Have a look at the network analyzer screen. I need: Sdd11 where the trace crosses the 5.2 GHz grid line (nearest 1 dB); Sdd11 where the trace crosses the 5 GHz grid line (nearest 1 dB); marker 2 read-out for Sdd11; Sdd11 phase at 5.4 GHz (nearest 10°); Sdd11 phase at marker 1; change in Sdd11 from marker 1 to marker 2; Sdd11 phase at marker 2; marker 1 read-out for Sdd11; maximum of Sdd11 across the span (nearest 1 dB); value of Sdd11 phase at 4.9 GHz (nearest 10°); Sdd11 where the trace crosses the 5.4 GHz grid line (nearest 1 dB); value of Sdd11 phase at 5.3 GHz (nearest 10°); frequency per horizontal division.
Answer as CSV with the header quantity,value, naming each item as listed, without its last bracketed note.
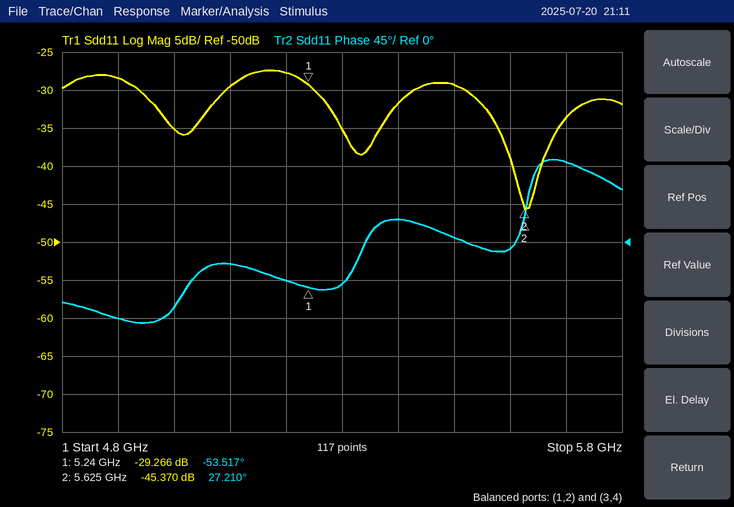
quantity,value
Sdd11 where the trace crosses the 5.2 GHz grid line,-28 dB
Sdd11 where the trace crosses the 5 GHz grid line,-35 dB
marker 2 read-out for Sdd11,-45.370 dB
Sdd11 phase at 5.4 GHz,30°
Sdd11 phase at marker 1,-53.517°
change in Sdd11 from marker 1 to marker 2,-16.104 dB
Sdd11 phase at marker 2,27.210°
marker 1 read-out for Sdd11,-29.266 dB
maximum of Sdd11 across the span,-27 dB
value of Sdd11 phase at 4.9 GHz,-90°
Sdd11 where the trace crosses the 5.4 GHz grid line,-32 dB
value of Sdd11 phase at 5.3 GHz,-50°
frequency per horizontal division,100 MHz
